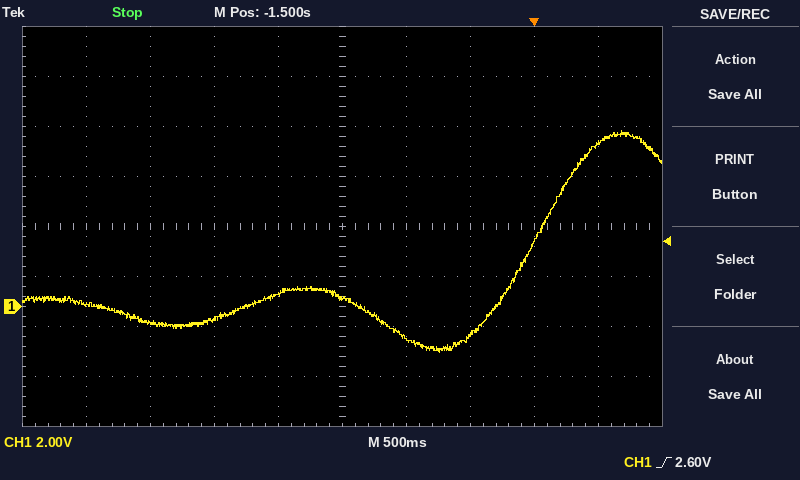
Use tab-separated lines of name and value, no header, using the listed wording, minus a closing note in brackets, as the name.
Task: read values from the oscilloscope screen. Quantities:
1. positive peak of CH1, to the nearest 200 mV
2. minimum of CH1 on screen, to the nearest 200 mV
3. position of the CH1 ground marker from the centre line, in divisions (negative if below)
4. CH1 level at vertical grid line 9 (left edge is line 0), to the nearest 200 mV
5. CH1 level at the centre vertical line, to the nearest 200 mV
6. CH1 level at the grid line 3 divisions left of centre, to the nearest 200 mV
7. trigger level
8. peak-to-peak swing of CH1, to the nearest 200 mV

positive peak of CH1, to the nearest 200 mV	7.0 V
minimum of CH1 on screen, to the nearest 200 mV	-1.8 V
position of the CH1 ground marker from the centre line, in divisions	-1.6 div
CH1 level at vertical grid line 9 (left edge is line 0), to the nearest 200 mV	6.4 V
CH1 level at the centre vertical line, to the nearest 200 mV	400 mV
CH1 level at the grid line 3 divisions left of centre, to the nearest 200 mV	-600 mV
trigger level	2.60 V
peak-to-peak swing of CH1, to the nearest 200 mV	8.8 V
